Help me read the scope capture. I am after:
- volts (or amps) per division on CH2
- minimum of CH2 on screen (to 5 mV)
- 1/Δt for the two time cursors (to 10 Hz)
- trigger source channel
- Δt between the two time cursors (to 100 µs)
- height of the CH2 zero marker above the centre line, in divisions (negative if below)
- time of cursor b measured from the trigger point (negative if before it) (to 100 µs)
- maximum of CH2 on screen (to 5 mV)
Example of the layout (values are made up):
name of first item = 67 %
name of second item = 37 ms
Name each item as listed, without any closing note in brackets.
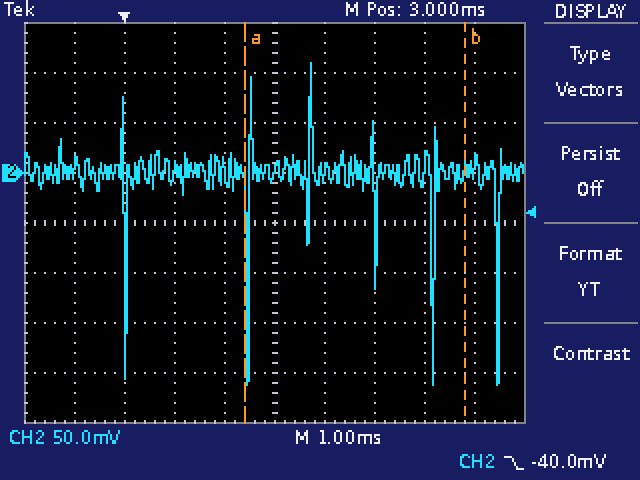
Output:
volts (or amps) per division on CH2 = 50 mV
minimum of CH2 on screen = -210 mV
1/Δt for the two time cursors = 230 Hz
trigger source channel = CH2
Δt between the two time cursors = 4.4 ms
height of the CH2 zero marker above the centre line, in divisions = +1.0 div
time of cursor b measured from the trigger point (negative if before it) = +6.8 ms
maximum of CH2 on screen = 110 mV
